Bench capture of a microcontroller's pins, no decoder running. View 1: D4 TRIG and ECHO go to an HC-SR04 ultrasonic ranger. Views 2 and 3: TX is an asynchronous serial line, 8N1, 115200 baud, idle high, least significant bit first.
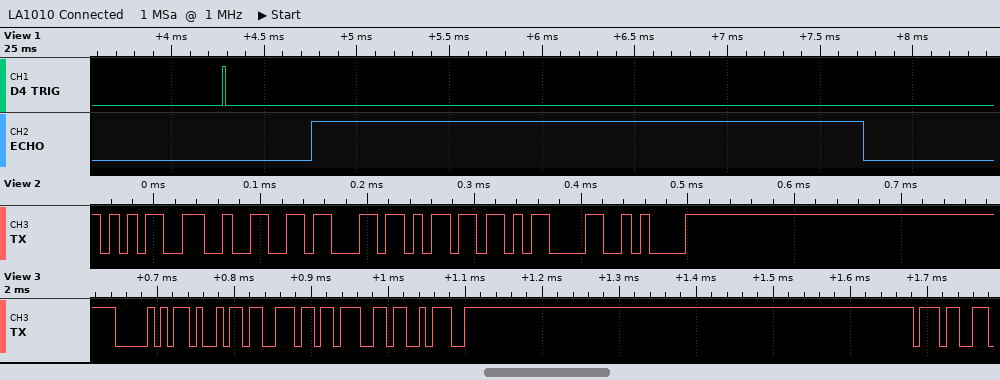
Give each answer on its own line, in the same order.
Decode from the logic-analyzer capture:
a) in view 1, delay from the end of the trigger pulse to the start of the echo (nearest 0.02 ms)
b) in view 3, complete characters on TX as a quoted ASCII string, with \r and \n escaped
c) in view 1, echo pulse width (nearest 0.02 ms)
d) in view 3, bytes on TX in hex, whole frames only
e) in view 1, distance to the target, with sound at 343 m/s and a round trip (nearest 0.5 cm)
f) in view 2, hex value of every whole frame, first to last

0.46 ms
"Ping:7"
2.98 ms
50 69 6E 67 3A 37
51 cm
0x35 0x32 0x63 0x6D 0x0D 0x0A
